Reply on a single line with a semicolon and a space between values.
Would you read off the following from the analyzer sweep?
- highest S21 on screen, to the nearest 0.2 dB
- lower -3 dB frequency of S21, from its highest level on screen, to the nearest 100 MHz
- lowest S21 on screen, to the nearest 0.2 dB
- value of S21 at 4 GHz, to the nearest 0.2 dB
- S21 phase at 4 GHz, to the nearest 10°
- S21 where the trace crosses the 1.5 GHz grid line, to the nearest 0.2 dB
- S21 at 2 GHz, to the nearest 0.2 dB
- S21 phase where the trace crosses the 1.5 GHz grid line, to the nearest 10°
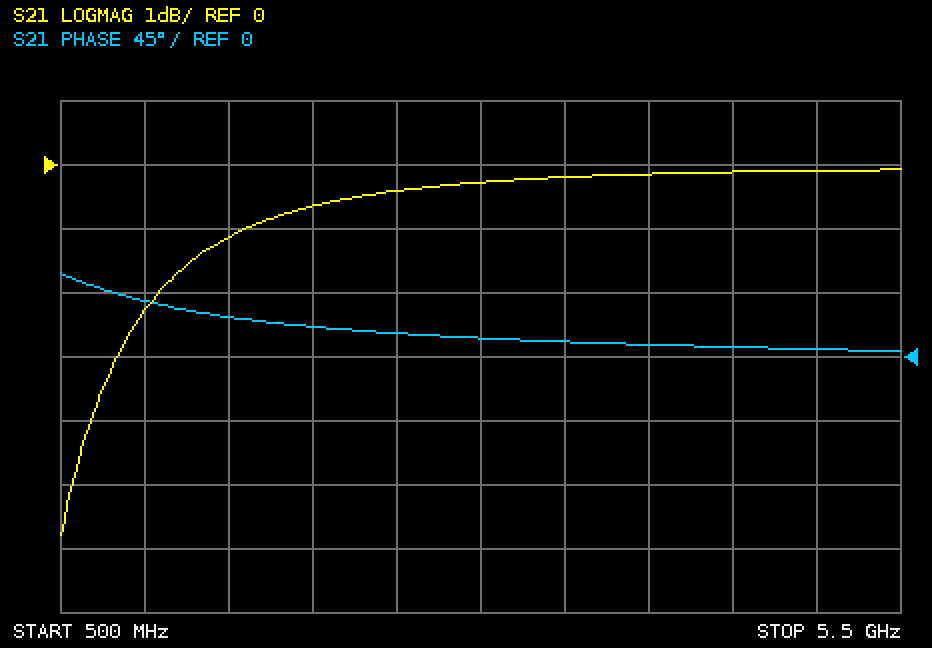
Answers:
0.0 dB; 800 MHz; -5.8 dB; -0.2 dB; 10°; -1.2 dB; -0.6 dB; 30°
